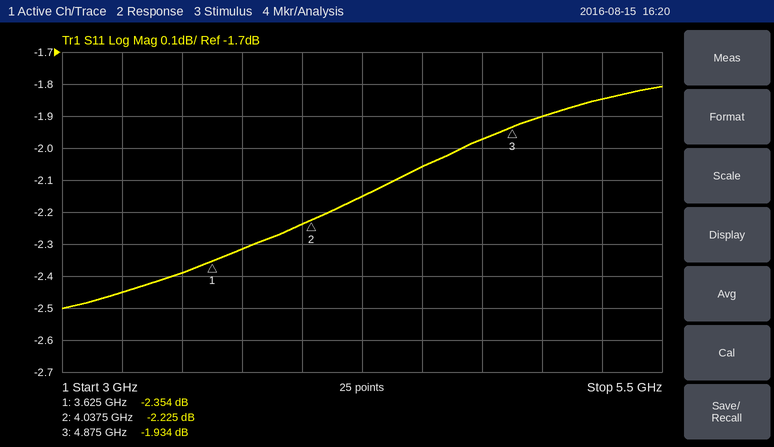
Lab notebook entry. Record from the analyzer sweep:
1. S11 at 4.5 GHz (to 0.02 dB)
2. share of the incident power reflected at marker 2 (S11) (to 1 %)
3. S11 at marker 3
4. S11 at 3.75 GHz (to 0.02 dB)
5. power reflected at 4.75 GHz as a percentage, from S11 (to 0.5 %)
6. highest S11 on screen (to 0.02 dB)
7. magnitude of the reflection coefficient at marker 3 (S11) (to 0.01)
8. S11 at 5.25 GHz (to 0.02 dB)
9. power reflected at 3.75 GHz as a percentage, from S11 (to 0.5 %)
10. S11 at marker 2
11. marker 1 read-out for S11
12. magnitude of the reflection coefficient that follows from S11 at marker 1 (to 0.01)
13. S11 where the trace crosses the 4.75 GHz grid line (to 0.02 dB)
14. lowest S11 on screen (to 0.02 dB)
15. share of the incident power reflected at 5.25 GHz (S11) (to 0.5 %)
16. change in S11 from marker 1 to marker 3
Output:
-2.06 dB
60 %
-1.934 dB
-2.32 dB
63.5 %
-1.80 dB
0.80
-1.84 dB
58.5 %
-2.225 dB
-2.354 dB
0.76
-1.98 dB
-2.50 dB
65.5 %
0.420 dB
